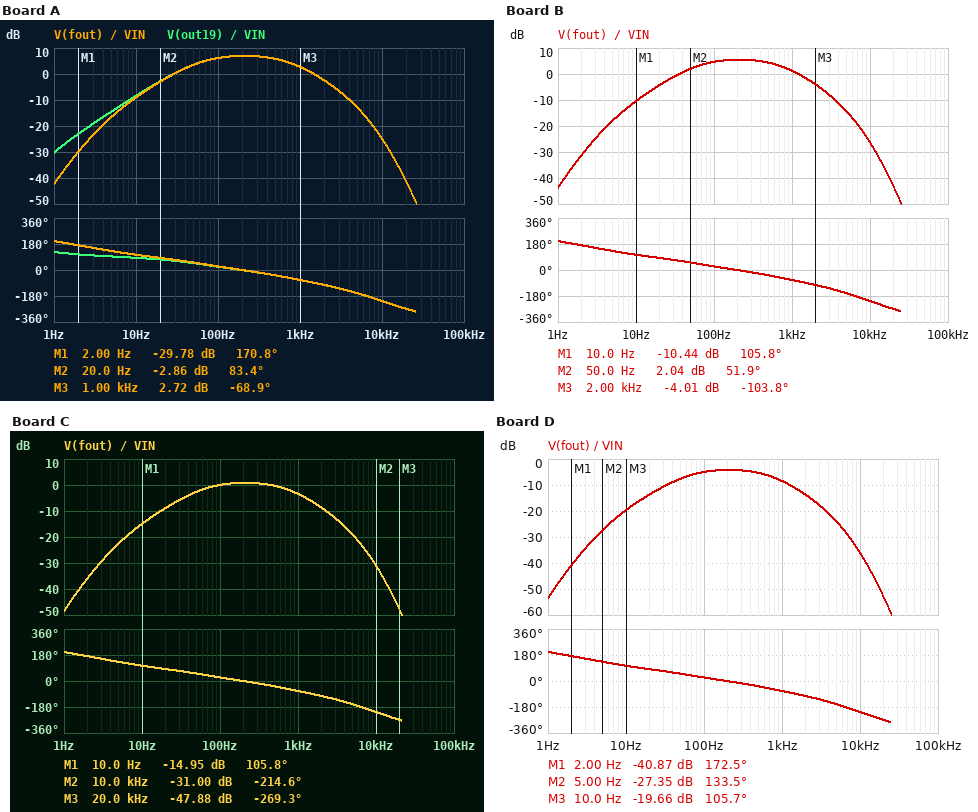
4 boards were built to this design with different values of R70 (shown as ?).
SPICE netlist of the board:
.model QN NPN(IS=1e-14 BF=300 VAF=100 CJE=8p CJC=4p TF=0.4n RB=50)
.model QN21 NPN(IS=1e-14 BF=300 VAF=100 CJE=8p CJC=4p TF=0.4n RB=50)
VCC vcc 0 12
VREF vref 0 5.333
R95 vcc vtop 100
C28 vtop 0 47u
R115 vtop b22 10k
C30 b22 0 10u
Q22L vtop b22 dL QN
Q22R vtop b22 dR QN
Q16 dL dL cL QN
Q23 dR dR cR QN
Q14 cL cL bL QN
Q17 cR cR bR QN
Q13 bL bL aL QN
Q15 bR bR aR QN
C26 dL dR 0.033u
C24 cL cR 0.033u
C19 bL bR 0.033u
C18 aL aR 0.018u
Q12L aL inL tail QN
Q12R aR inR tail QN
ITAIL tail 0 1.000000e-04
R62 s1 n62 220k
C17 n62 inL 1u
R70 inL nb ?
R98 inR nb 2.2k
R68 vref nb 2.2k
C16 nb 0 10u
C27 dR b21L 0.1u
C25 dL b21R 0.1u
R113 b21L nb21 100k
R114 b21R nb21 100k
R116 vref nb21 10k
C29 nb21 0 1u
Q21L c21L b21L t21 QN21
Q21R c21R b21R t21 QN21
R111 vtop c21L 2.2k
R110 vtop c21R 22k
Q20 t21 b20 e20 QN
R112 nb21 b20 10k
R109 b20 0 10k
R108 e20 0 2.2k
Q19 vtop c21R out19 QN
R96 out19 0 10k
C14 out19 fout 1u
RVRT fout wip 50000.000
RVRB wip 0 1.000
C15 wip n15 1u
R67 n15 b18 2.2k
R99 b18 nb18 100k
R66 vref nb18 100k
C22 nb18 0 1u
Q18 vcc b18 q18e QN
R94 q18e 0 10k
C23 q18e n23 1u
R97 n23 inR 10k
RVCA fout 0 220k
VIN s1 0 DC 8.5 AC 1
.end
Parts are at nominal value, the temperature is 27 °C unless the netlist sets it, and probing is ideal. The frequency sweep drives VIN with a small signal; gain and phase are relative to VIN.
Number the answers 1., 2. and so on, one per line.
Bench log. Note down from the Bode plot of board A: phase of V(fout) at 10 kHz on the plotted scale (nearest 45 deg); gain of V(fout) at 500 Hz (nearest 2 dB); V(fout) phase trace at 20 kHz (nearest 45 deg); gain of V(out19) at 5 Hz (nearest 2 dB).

1. -225 deg
2. 6 dB
3. -270 deg
4. -14 dB
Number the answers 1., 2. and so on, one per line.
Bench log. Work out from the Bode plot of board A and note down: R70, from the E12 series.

1. 5.6 kΩ
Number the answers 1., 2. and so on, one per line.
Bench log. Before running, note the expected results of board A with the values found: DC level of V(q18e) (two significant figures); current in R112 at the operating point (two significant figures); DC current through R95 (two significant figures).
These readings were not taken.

1. 4.4 V
2. 180 µA
3. 1.2 mA
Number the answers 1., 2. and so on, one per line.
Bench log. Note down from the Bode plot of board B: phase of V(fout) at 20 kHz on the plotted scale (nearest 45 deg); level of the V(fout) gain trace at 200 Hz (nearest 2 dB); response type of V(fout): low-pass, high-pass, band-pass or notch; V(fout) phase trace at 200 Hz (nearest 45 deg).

1. -270 deg
2. 6 dB
3. band-pass
4. 0 deg
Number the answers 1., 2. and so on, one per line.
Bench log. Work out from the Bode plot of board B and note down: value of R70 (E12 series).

1. 4.7 kΩ
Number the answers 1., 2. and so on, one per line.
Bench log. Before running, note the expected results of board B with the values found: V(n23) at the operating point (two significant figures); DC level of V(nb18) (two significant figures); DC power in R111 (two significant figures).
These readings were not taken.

1. 5.3 V
2. 5.2 V
3. 150 µW
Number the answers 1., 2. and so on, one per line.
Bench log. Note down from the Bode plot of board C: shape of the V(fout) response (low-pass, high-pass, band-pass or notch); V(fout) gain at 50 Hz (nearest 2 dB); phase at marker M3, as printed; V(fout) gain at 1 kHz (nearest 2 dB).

1. band-pass
2. -2 dB
3. -269.3 deg
4. -4 dB
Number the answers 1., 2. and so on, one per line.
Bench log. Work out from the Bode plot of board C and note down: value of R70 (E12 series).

1. 2.7 kΩ
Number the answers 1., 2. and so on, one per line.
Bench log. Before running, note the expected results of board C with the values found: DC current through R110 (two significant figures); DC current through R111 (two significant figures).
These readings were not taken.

1. 250 µA
2. 260 µA
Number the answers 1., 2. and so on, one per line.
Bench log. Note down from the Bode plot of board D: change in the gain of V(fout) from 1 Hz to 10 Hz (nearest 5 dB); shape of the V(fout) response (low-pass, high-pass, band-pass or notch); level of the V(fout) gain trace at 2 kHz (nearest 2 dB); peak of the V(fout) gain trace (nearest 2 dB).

1. 35 dB
2. band-pass
3. -14 dB
4. -4 dB
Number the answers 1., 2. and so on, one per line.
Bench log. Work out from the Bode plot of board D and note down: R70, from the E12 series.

1. 1.5 kΩ
